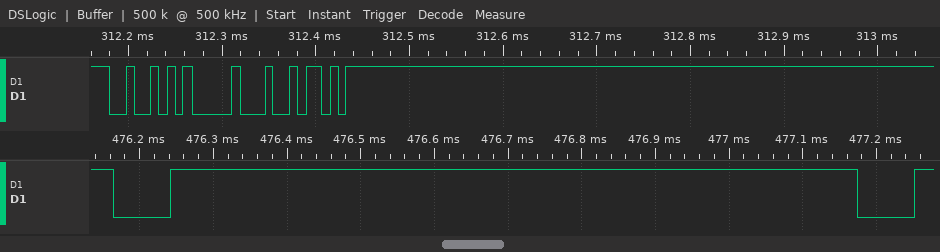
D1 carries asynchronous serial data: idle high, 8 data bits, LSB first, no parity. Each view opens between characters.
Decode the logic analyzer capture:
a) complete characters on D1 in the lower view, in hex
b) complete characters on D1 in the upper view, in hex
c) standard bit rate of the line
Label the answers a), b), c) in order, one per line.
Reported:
a) 00, 00
b) 52, 10, 5A
c) 115200 baud
